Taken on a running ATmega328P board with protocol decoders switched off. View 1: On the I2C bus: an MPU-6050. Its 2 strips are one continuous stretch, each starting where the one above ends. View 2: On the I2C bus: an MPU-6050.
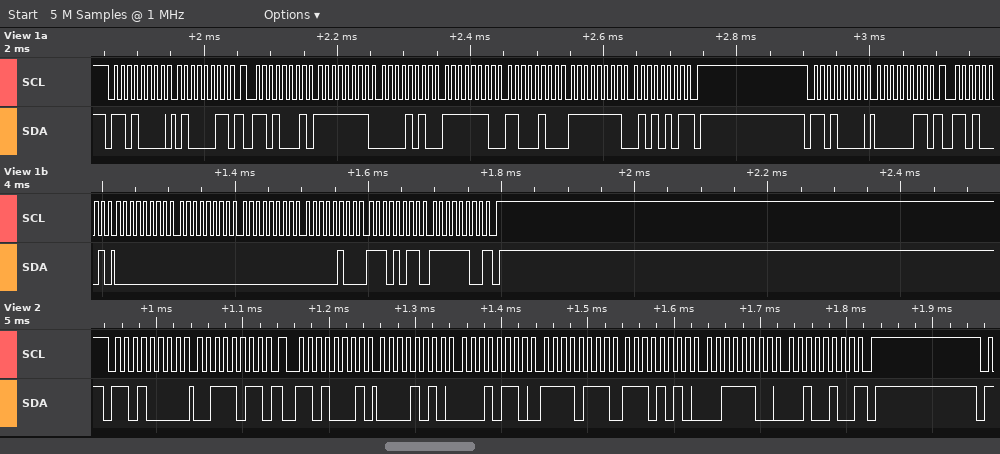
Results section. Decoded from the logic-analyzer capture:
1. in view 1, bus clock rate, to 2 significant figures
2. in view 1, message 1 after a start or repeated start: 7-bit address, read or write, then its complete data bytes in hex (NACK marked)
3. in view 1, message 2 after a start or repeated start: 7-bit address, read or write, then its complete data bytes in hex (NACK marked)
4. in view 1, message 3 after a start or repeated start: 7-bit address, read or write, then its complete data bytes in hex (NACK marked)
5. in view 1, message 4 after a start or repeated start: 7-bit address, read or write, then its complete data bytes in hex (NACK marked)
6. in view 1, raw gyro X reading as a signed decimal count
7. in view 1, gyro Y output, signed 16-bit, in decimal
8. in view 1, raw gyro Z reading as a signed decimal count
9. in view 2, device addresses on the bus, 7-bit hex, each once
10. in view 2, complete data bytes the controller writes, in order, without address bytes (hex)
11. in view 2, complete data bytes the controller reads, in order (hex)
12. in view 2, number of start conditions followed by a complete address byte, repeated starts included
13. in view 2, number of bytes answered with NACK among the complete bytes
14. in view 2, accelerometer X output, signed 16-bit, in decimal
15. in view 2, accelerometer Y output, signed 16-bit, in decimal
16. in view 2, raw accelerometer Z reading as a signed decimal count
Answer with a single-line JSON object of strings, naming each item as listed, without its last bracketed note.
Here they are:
{"in view 1, bus clock rate, to 2 significant figures": "100 kHz", "in view 1, message 1 after a start or repeated start: 7-bit address, read or write, then its complete data bytes in hex": "0x68 write: 43", "in view 1, message 2 after a start or repeated start: 7-bit address, read or write, then its complete data bytes in hex": "0x68 read: FF 0A FE C4 FF 55 NACK", "in view 1, message 3 after a start or repeated start: 7-bit address, read or write, then its complete data bytes in hex": "0x68 write: 03", "in view 1, message 4 after a start or repeated start: 7-bit address, read or write, then its complete data bytes in hex": "0x68 read: 00 00 00 04 EB FC NACK", "in view 1, raw gyro X reading as a signed decimal count": "-246", "in view 1, gyro Y output, signed 16-bit, in decimal": "-316", "in view 1, raw gyro Z reading as a signed decimal count": "-171", "in view 2, device addresses on the bus, 7-bit hex, each once": "0x68", "in view 2, complete data bytes the controller writes, in order, without address bytes": "3B", "in view 2, complete data bytes the controller reads, in order": "0A 16 F7 EA 3C 24", "in view 2, number of start conditions followed by a complete address byte, repeated starts included": "2", "in view 2, number of bytes answered with NACK among the complete bytes": "1", "in view 2, accelerometer X output, signed 16-bit, in decimal": "2582", "in view 2, accelerometer Y output, signed 16-bit, in decimal": "-2070", "in view 2, raw accelerometer Z reading as a signed decimal count": "15396"}
